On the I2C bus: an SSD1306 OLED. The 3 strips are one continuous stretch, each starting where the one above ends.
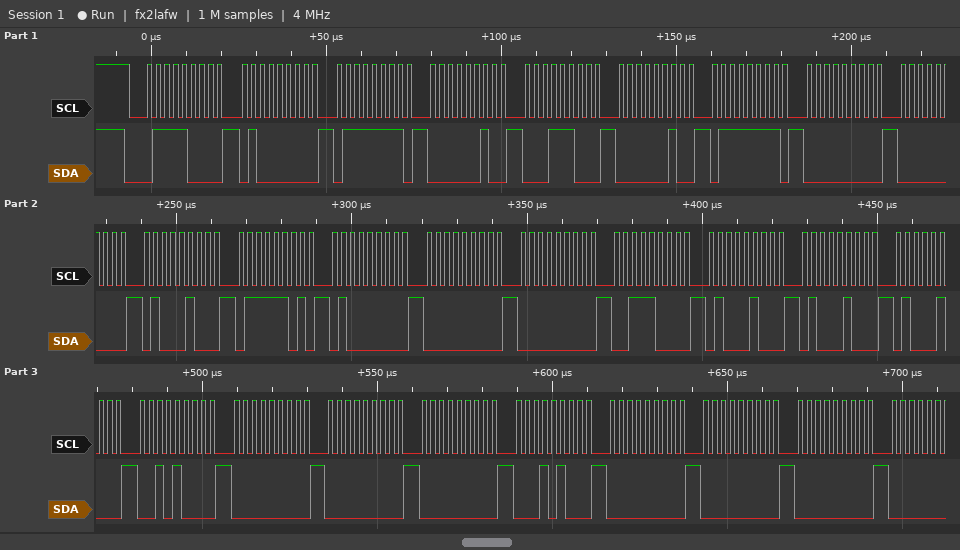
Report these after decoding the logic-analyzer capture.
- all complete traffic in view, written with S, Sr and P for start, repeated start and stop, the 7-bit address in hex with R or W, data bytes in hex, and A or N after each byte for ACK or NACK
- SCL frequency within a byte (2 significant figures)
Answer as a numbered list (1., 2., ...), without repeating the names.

1. S 3CW A 40 A 7F A 02 A 1C A 02 A 7F A 00 A 00 A 44 A 7D A 40 A 00 A 00 A 38 A 44 A 44 A 44 A 28 A 00 A 00 A 00 A 14 A 00 A 00 A 00 A
2. 400 kHz
